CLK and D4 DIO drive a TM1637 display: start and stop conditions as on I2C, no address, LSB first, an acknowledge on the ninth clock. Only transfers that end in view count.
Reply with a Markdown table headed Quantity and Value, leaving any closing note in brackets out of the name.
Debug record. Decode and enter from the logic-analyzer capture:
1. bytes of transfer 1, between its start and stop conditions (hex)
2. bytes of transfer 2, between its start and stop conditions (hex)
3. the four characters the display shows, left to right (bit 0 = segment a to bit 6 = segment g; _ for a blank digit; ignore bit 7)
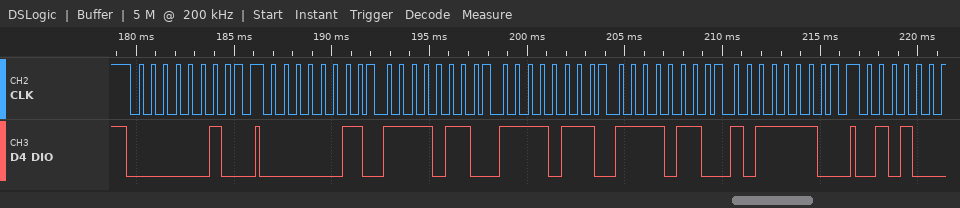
| Quantity | Value |
|---|---|
| bytes of transfer 1, between its start and stop conditions | 40 |
| bytes of transfer 2, between its start and stop conditions | C0 6F EF 6F 7D |
| the four characters the display shows, left to right | 9996 |
